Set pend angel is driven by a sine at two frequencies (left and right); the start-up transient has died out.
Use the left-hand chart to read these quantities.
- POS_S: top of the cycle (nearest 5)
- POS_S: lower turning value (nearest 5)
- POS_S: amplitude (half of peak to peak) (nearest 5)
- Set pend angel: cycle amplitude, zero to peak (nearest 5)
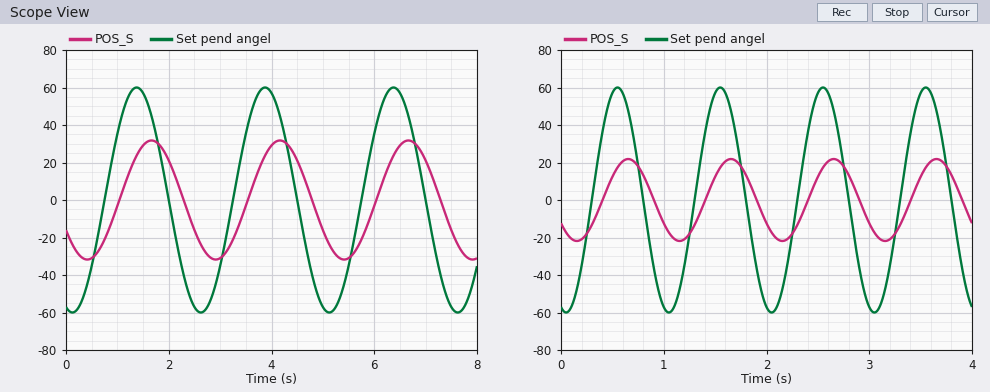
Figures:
30
-30
30
60
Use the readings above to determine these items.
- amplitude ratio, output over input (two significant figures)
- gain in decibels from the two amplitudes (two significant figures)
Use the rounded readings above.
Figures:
0.50
-6.0 dB
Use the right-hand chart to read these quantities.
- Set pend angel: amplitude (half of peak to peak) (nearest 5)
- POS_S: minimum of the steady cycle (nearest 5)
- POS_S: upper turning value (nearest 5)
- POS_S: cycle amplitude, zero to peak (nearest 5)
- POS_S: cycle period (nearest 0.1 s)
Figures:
60
-20
20
20
1.0 s
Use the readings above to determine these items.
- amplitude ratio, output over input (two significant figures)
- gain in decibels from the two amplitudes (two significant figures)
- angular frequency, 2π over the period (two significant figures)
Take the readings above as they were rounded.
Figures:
0.33
-9.5 dB
6.3 rad/s
